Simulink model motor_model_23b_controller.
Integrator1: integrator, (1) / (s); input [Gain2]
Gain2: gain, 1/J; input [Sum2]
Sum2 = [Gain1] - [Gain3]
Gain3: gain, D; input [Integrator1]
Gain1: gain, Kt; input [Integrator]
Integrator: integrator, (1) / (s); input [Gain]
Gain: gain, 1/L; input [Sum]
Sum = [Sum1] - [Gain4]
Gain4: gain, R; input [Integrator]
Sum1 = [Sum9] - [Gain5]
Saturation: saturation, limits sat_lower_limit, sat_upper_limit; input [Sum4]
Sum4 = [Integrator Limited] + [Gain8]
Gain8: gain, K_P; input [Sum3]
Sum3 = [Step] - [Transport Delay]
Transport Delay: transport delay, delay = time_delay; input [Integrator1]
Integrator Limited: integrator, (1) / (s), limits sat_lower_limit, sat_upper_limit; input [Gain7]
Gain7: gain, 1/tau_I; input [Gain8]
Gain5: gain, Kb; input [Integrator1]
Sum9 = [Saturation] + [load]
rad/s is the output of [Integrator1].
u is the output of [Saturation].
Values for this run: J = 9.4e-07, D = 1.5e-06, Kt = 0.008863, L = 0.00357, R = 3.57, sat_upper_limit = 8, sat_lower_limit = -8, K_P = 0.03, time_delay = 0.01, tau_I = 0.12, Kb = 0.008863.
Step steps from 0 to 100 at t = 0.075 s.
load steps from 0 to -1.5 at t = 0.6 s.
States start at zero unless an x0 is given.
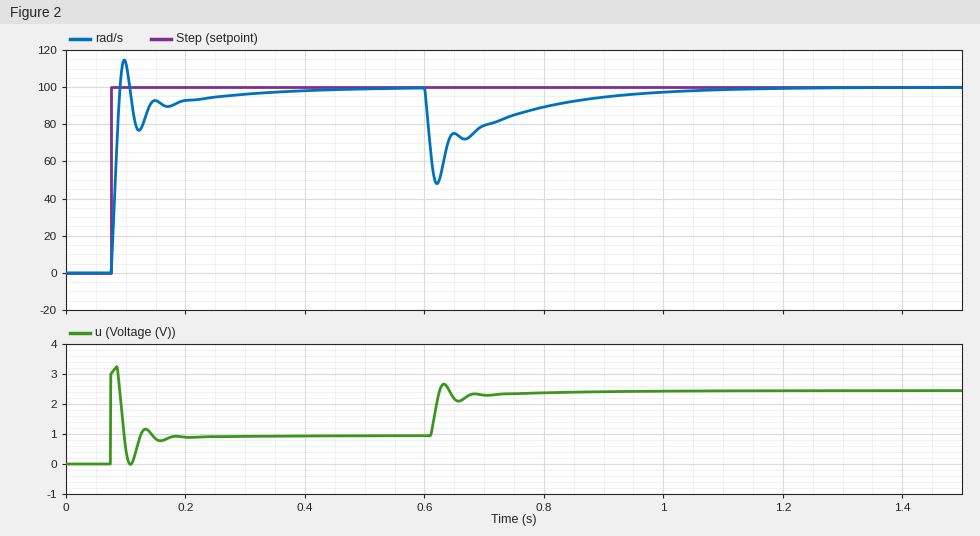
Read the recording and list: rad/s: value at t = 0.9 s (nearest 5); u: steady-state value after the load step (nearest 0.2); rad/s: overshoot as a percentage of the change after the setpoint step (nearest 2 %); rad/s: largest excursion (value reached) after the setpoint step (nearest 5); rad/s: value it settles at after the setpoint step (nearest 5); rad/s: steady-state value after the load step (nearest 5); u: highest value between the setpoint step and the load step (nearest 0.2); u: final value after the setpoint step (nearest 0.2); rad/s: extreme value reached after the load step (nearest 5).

95
2.4
14 %
115
100
100
3.2
1.0
50
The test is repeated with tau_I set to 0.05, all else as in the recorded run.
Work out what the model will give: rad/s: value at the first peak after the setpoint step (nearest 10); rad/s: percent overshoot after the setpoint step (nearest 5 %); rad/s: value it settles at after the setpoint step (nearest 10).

130
30 %
100
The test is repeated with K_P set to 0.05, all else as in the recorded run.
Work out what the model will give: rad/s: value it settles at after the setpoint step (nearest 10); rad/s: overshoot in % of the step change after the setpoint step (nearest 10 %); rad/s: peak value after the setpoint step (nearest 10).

100
70 %
170
